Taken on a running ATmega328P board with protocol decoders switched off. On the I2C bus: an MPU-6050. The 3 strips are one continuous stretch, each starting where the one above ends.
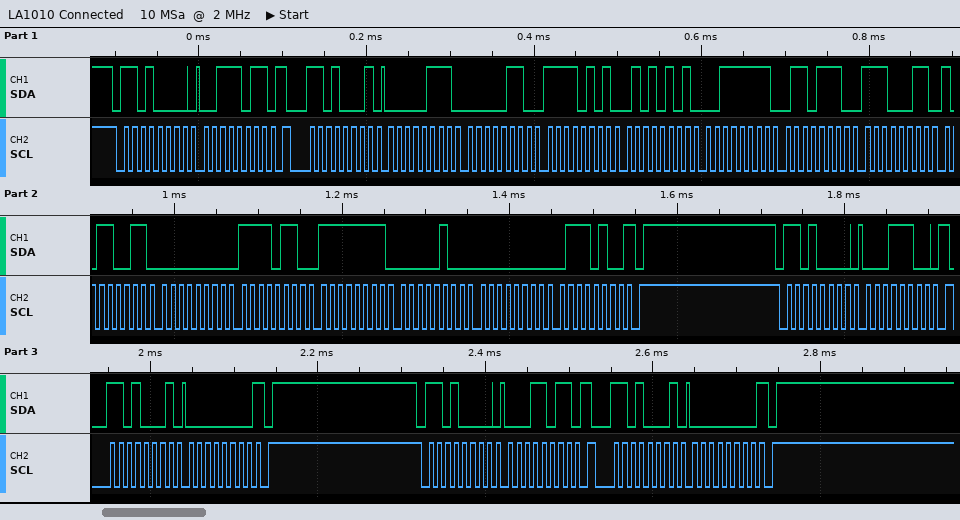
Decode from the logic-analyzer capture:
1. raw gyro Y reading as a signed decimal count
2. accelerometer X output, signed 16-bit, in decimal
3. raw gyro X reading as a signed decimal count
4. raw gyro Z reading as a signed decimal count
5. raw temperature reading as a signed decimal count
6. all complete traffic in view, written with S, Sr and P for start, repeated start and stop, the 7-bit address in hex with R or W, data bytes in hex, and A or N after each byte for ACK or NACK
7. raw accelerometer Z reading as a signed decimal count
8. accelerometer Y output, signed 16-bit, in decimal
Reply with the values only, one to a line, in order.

-252
1798
246
116
-7245
S 68W A 3B A Sr 68R A 07 A 06 A F5 A 55 A 3F A 6E A E3 A B3 A 00 A F6 A FF A 04 A 00 A 74 N P S 68W A 1C A Sr 68R A 00 N P S 68W A 1B A Sr 68R A 00 N P
16238
-2731
